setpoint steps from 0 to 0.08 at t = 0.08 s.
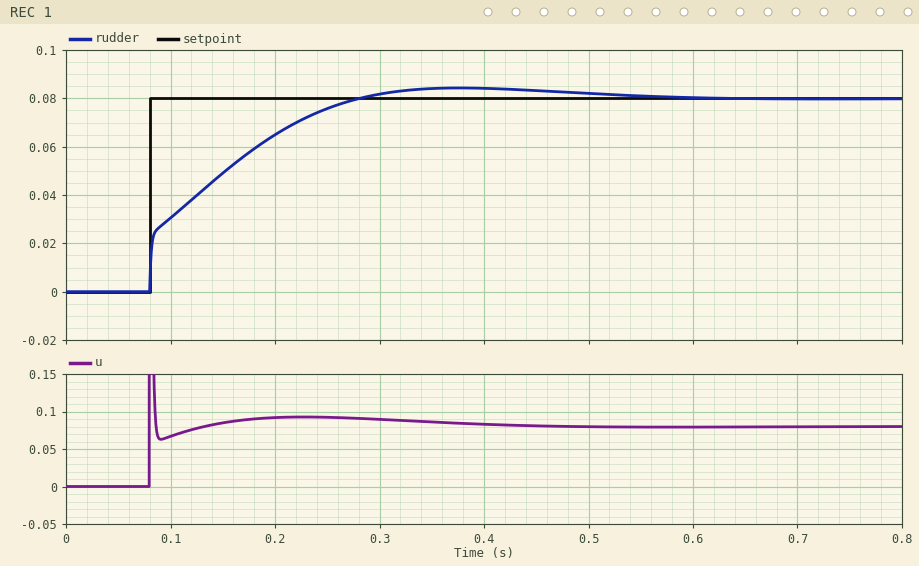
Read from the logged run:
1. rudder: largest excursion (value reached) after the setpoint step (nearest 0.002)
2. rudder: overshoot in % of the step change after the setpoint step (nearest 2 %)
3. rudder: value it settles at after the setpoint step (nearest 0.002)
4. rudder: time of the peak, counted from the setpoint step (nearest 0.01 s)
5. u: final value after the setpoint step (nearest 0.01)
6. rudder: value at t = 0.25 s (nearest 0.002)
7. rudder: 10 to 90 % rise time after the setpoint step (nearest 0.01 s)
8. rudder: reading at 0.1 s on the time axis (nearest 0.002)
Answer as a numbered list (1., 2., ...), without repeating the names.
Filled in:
1. 0.084
2. 6 %
3. 0.080
4. 0.30 s
5. 0.08
6. 0.076
7. 0.15 s
8. 0.030
